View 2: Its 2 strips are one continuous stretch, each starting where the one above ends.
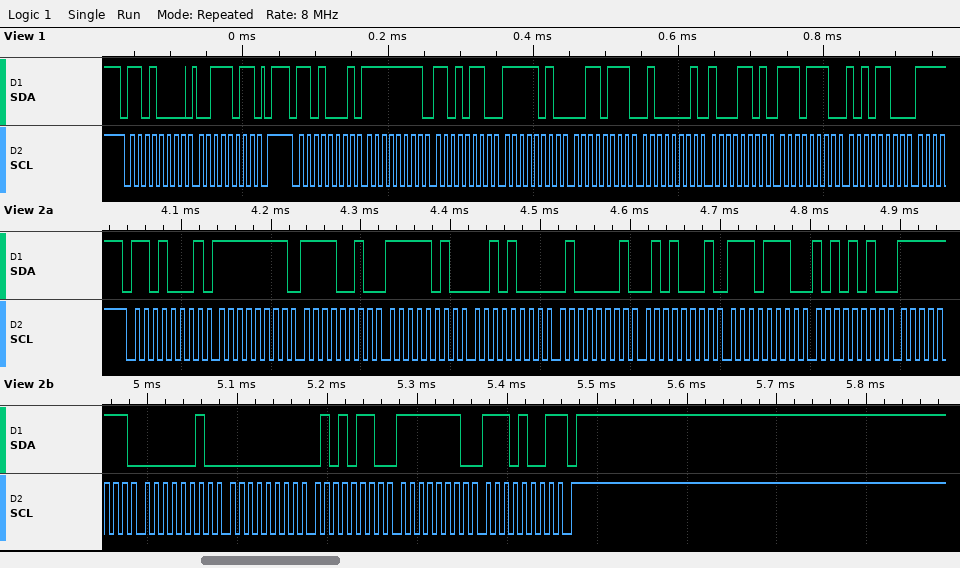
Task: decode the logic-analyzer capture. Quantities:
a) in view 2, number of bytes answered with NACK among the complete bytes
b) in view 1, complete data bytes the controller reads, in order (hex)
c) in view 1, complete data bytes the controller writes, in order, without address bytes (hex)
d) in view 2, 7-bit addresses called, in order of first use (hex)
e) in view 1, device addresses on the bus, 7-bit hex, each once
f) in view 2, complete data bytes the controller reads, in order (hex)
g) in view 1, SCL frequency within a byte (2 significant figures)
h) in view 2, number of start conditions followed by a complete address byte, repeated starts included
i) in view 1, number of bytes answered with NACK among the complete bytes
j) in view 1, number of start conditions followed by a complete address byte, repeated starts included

1
FF D6 FA 37 41 8D EE AC
3B
0x68
0x68
FF F2 FA 28 41 51 EE AA FF 02 00 56 FE E9
100 kHz
1
0
2
